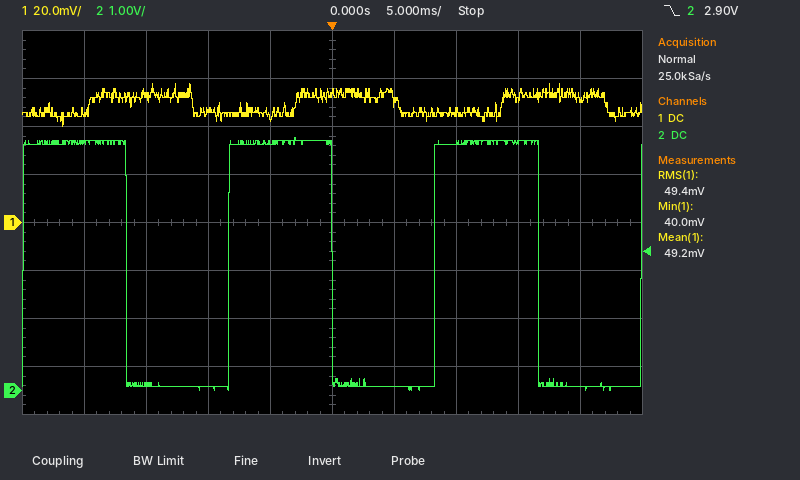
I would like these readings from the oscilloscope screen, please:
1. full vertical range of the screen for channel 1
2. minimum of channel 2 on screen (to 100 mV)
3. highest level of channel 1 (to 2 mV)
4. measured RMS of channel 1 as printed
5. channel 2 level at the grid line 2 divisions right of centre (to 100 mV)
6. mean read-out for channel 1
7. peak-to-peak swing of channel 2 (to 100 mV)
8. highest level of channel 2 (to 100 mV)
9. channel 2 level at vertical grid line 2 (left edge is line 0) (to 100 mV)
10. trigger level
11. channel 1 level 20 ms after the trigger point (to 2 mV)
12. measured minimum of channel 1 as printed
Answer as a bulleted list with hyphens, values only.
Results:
- 160 mV
- 0.0 V
- 58 mV
- 49.4 mV
- 5.2 V
- 49.2 mV
- 5.3 V
- 5.3 V
- 100 mV
- 2.90 V
- 52 mV
- 40.0 mV
